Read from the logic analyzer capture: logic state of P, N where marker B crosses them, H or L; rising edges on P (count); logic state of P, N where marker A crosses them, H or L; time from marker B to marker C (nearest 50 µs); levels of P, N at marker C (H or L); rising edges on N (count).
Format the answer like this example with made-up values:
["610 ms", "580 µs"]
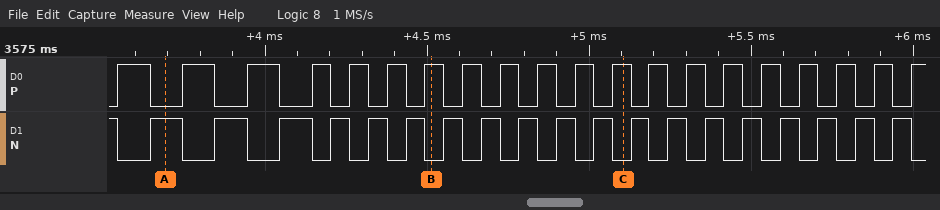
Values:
["P=H, N=L", "20", "P=L, N=H", "600 µs", "P=H, N=L", "19"]
